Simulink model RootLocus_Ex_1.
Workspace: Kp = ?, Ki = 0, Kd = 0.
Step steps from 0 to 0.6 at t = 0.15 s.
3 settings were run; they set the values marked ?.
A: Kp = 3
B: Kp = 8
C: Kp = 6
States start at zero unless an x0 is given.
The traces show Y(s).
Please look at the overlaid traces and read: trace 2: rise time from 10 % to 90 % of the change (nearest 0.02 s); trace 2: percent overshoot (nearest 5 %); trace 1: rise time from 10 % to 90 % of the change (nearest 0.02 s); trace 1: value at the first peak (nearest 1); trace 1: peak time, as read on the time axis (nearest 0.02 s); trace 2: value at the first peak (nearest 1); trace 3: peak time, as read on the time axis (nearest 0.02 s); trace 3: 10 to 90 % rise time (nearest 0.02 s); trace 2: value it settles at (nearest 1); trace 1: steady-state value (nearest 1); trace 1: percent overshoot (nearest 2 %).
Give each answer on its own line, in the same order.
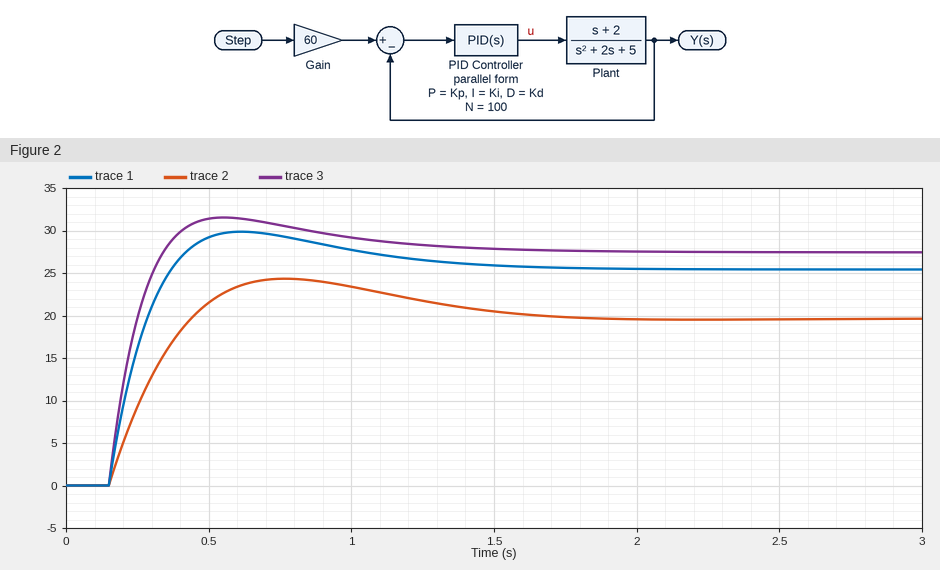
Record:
0.22 s
25 %
0.16 s
30
0.62 s
24
0.56 s
0.14 s
20
25
18 %
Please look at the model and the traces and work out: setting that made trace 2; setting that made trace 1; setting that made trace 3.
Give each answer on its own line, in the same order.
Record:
A
C
B
